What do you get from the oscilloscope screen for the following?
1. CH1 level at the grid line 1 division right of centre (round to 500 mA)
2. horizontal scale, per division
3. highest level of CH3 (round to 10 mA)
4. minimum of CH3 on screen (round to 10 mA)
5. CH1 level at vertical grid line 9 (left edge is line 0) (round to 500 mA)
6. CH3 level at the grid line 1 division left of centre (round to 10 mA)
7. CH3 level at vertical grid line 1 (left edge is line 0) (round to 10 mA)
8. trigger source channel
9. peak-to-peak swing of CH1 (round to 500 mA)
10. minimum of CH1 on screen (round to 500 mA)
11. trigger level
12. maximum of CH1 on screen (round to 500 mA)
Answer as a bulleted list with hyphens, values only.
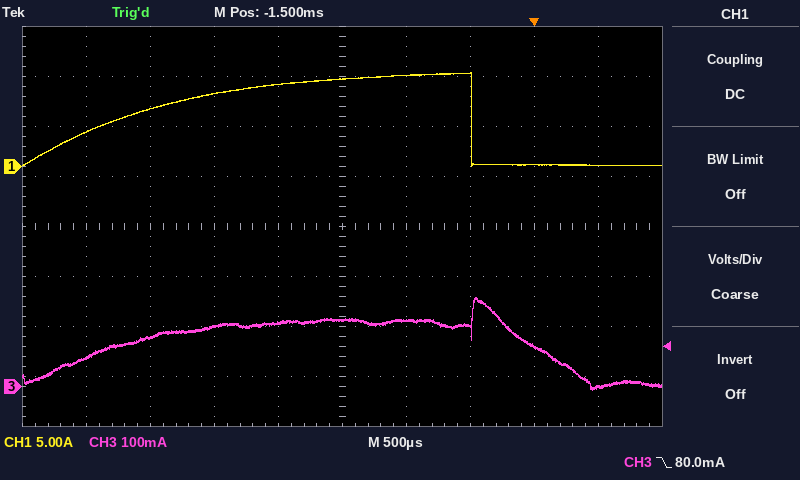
- 9.0 A
- 500 µs
- 180 mA
- -10 mA
- 0.0 A
- 130 mA
- 60 mA
- CH3
- 9.5 A
- 0.0 A
- 80.0 mA
- 9.5 A
